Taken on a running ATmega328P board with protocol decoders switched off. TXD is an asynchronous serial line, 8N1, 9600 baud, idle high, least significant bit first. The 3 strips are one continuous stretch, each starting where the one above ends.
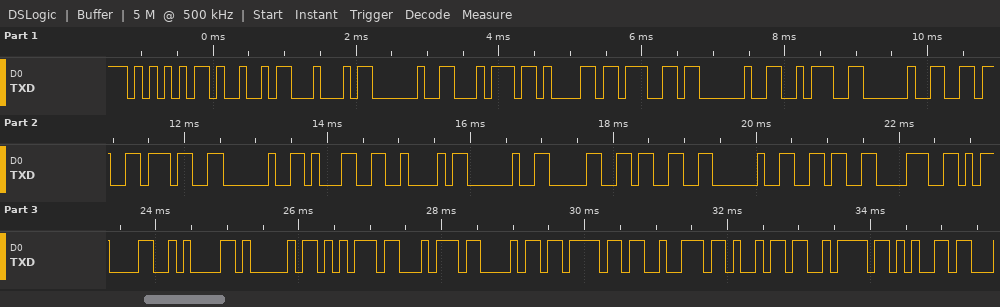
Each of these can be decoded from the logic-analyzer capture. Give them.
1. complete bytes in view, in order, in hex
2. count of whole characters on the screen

55 49 44 20 74 61 67 20 3A 20 36 37 20 31 42 20 30 33 20 36 38 0D 0A 41 75 74 68 6F 72 69 7A 65
32
